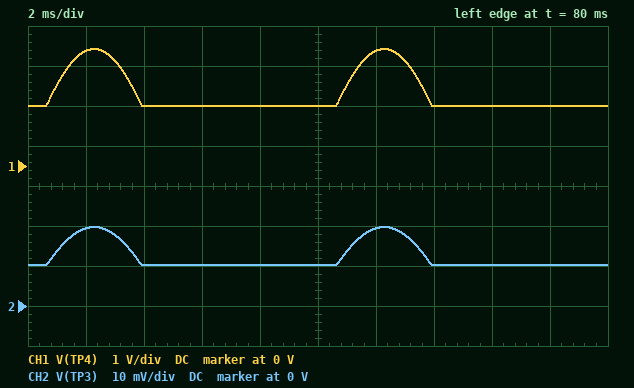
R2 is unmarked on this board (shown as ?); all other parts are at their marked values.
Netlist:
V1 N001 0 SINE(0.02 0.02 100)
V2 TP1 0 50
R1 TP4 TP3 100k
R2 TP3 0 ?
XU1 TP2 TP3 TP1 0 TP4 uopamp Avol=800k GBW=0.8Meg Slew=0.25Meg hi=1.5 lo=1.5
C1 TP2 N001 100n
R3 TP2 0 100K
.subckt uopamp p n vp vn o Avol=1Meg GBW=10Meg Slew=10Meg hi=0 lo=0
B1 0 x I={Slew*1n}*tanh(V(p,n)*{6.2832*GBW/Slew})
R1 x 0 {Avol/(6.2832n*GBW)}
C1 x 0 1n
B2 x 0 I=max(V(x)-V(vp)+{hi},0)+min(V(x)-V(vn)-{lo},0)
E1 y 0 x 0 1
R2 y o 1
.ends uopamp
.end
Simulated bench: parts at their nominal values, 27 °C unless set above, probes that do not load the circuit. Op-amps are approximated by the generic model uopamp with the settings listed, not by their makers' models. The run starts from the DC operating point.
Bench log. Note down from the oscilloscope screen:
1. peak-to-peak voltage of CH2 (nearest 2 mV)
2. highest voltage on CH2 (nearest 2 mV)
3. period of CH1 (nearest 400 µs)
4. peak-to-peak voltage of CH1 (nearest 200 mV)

10 mV
20 mV
10.0 ms
1.4 V
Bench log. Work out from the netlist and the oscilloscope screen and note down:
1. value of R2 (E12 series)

680 Ω
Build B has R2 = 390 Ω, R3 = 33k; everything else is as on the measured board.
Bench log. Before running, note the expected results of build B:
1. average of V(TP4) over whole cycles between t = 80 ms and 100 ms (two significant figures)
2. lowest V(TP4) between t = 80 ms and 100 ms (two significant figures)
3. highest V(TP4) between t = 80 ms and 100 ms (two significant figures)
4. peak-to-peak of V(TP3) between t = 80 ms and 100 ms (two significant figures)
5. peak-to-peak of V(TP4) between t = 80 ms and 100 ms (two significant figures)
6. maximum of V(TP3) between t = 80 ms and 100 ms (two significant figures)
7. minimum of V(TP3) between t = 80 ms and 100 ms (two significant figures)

2.3 V
1.5 V
4.6 V
12 mV
3.1 V
18 mV
5.8 mV
